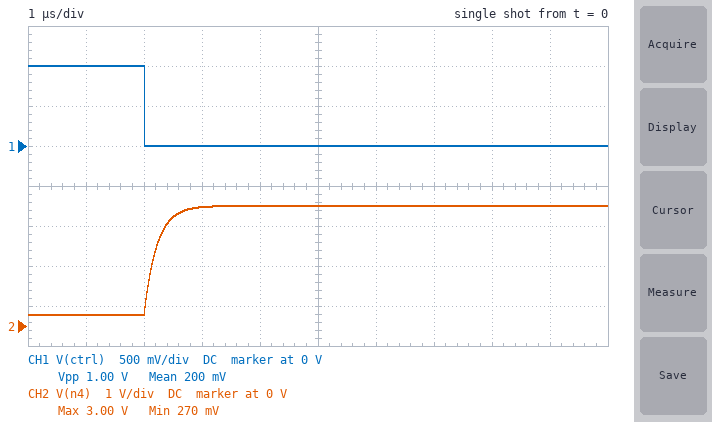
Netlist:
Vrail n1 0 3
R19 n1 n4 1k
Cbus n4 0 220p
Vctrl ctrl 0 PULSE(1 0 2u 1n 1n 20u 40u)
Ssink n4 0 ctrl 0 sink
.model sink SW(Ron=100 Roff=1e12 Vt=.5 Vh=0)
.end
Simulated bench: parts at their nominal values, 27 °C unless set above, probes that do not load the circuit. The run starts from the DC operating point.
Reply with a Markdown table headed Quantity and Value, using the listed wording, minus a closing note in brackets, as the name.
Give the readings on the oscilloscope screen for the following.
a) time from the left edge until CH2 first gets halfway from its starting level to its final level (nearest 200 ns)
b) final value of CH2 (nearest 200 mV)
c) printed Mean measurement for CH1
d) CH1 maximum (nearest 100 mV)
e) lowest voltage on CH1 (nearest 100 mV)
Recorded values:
| Quantity | Value |
|---|---|
| time from the left edge until CH2 first gets halfway from its starting level to its final level | 2.2 µs |
| final value of CH2 | 3.0 V |
| printed Mean measurement for CH1 | 200 mV |
| CH1 maximum | 1.0 V |
| lowest voltage on CH1 | 0 V |
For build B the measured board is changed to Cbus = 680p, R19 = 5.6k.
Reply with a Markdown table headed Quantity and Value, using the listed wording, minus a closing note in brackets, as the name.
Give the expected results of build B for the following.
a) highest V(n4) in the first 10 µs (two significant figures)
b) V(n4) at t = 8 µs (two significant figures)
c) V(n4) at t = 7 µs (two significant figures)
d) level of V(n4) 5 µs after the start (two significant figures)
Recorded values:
| Quantity | Value |
|---|---|
| highest V(n4) in the first 10 µs | 2.6 V |
| V(n4) at t = 8 µs | 2.4 V |
| V(n4) at t = 7 µs | 2.2 V |
| level of V(n4) 5 µs after the start | 1.7 V |
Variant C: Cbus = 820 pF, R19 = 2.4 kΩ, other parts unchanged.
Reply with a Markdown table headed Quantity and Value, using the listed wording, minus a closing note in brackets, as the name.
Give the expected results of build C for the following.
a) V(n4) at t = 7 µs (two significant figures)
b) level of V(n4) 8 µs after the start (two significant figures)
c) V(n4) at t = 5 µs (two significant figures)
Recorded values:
| Quantity | Value |
|---|---|
| V(n4) at t = 7 µs | 2.8 V |
| level of V(n4) 8 µs after the start | 2.9 V |
| V(n4) at t = 5 µs | 2.4 V |
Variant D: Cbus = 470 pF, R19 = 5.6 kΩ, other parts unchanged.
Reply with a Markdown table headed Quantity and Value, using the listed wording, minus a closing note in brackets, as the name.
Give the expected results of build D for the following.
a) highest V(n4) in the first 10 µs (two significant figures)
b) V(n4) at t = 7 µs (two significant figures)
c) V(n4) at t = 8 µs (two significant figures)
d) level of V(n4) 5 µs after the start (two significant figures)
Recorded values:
| Quantity | Value |
|---|---|
| highest V(n4) in the first 10 µs | 2.9 V |
| V(n4) at t = 7 µs | 2.6 V |
| V(n4) at t = 8 µs | 2.7 V |
| level of V(n4) 5 µs after the start | 2.1 V |
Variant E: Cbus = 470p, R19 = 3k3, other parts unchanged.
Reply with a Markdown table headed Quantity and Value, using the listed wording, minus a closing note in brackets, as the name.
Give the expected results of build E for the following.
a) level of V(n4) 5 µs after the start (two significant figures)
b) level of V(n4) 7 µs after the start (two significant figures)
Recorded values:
| Quantity | Value |
|---|---|
| level of V(n4) 5 µs after the start | 2.6 V |
| level of V(n4) 7 µs after the start | 2.9 V |
